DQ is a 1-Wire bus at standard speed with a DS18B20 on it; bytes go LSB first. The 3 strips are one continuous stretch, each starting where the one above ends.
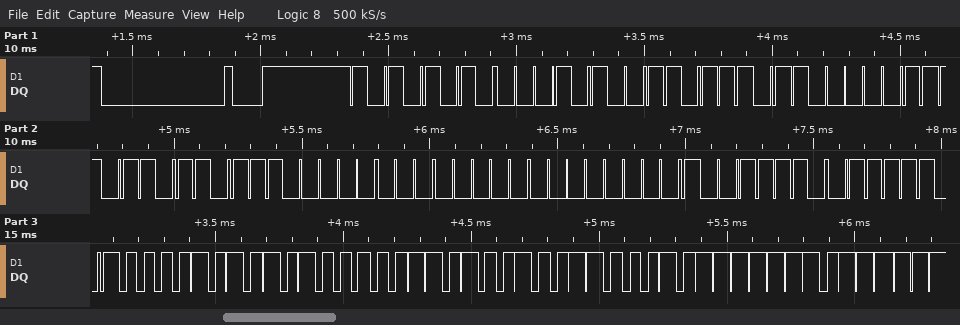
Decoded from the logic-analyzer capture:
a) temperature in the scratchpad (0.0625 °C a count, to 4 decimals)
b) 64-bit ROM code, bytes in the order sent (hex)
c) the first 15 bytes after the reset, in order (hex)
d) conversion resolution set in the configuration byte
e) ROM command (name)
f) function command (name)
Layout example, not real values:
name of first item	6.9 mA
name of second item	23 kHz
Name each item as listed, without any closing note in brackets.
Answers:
temperature in the scratchpad	85.0000 °C
64-bit ROM code, bytes in the order sent	28 BB C1 6D 07 00 00 79
the first 15 bytes after the reset, in order	55 28 BB C1 6D 07 00 00 79 BE 50 05 4B 46 7F
conversion resolution set in the configuration byte	12 bits
ROM command	Match ROM
function command	Read Scratchpad
